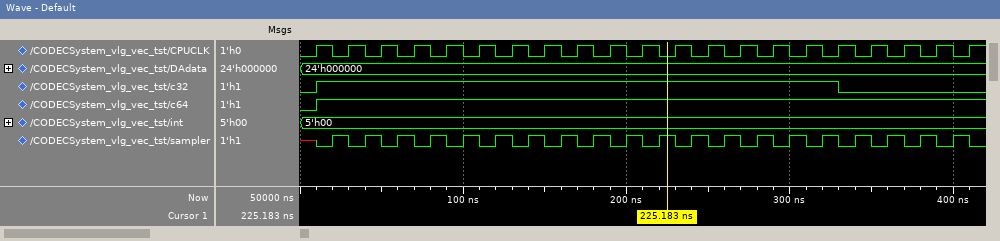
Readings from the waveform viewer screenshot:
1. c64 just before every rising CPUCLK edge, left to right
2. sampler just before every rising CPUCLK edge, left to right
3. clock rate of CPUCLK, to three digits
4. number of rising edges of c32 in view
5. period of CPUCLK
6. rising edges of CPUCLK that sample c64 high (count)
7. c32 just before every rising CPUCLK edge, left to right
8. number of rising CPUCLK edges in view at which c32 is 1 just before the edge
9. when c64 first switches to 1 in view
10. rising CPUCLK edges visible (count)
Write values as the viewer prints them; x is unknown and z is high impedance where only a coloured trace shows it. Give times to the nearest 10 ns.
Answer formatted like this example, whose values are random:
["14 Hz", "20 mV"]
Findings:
["0 1 1 1 1 1 1 1 1 1 1 1 1 1 1 1 1 1 1 1 1", "x 1 1 1 1 1 1 1 1 1 1 1 1 1 1 1 1 1 1 1 1", "50.0 MHz", "1", "20 ns", "20", "0 1 1 1 1 1 1 1 1 1 1 1 1 1 1 1 1 0 0 0 0", "16", "10 ns", "21"]
